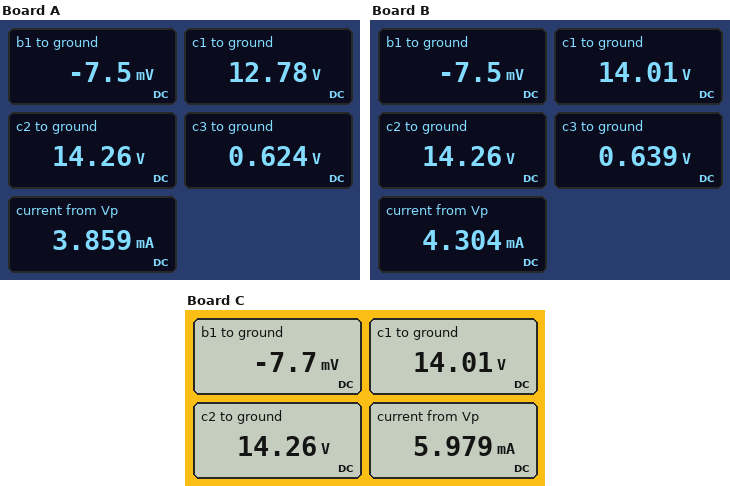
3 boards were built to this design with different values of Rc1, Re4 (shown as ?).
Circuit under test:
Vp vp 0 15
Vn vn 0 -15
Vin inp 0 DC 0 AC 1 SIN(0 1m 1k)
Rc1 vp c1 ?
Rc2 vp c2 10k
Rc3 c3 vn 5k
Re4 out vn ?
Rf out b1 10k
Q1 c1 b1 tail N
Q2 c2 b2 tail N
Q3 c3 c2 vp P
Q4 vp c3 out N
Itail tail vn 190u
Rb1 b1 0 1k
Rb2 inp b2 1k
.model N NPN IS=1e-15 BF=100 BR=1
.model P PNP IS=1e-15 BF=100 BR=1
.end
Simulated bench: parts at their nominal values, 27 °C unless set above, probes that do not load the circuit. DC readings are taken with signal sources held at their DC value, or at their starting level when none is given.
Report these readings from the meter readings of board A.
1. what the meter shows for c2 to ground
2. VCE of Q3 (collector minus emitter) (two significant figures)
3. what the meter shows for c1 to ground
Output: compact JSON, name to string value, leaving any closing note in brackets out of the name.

{"what the meter shows for c2 to ground": "14.26 V", "VCE of Q3 (collector minus emitter)": "-14 V", "what the meter shows for c1 to ground": "12.78 V"}
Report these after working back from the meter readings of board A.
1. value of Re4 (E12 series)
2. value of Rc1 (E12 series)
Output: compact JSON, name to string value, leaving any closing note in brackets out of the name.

{"value of Re4": "27 kΩ", "value of Rc1": "27 kΩ"}
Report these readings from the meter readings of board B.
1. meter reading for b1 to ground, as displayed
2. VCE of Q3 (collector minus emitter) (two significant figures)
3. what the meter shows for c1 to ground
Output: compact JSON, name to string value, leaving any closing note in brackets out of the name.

{"meter reading for b1 to ground, as displayed": "-7.5 mV", "VCE of Q3 (collector minus emitter)": "-14 V", "what the meter shows for c1 to ground": "14.01 V"}
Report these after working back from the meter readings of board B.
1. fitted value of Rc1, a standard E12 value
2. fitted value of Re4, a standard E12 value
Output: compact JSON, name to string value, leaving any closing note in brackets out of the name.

{"fitted value of Rc1, a standard E12 value": "12 kΩ", "fitted value of Re4, a standard E12 value": "15 kΩ"}
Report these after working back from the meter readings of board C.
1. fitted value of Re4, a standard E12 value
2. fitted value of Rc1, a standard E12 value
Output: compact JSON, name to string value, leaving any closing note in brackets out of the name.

{"fitted value of Re4, a standard E12 value": "5.6 kΩ", "fitted value of Rc1, a standard E12 value": "12 kΩ"}
